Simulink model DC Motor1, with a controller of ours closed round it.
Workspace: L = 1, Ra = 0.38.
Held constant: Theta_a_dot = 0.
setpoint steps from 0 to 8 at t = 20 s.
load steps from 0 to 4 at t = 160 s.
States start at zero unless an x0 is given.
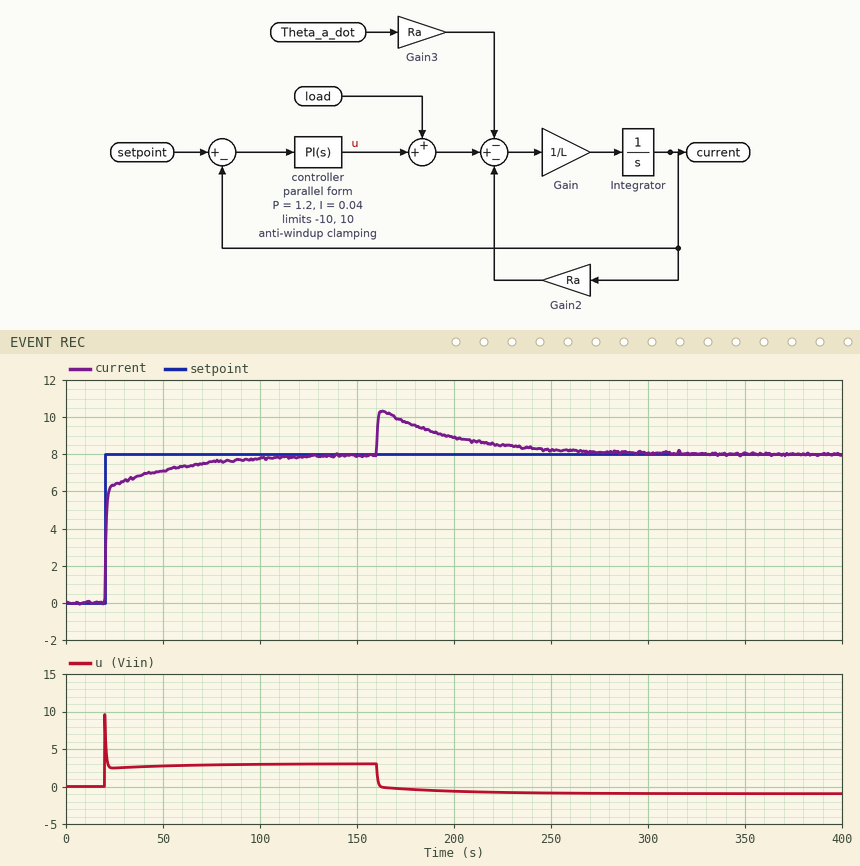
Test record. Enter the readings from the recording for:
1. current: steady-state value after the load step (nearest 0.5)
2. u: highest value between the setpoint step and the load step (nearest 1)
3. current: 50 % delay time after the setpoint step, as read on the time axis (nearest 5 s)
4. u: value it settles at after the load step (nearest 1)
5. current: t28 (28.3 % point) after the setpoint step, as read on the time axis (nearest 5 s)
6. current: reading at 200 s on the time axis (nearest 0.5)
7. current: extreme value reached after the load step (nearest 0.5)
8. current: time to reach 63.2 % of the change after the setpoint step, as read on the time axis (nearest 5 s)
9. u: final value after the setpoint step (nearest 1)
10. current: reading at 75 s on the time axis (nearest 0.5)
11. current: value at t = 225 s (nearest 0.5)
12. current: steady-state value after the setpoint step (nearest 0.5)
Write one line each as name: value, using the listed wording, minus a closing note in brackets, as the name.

current: steady-state value after the load step: 8.0
u: highest value between the setpoint step and the load step: 10
current: 50 % delay time after the setpoint step, as read on the time axis: 20 s
u: value it settles at after the load step: -1
current: t28 (28.3 % point) after the setpoint step, as read on the time axis: 20 s
current: reading at 200 s on the time axis: 9.0
current: extreme value reached after the load step: 10.5
current: time to reach 63.2 % of the change after the setpoint step, as read on the time axis: 20 s
u: final value after the setpoint step: 3
current: reading at 75 s on the time axis: 7.5
current: value at t = 225 s: 8.5
current: steady-state value after the setpoint step: 8.0
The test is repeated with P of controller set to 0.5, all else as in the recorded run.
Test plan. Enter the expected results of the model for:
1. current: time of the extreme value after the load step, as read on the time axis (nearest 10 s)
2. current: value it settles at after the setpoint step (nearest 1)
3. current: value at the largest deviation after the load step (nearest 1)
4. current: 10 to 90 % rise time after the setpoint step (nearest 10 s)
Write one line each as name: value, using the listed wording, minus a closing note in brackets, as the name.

current: time of the extreme value after the load step, as read on the time axis: 160 s
current: value it settles at after the setpoint step: 8
current: value at the largest deviation after the load step: 12
current: 10 to 90 % rise time after the setpoint step: 30 s
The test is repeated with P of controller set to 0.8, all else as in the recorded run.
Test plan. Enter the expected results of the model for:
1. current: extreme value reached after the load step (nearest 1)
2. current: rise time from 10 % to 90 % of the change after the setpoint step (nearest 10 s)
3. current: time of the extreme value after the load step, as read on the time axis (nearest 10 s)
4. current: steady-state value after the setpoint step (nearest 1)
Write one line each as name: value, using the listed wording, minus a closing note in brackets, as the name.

current: extreme value reached after the load step: 11
current: rise time from 10 % to 90 % of the change after the setpoint step: 30 s
current: time of the extreme value after the load step, as read on the time axis: 160 s
current: steady-state value after the setpoint step: 8
